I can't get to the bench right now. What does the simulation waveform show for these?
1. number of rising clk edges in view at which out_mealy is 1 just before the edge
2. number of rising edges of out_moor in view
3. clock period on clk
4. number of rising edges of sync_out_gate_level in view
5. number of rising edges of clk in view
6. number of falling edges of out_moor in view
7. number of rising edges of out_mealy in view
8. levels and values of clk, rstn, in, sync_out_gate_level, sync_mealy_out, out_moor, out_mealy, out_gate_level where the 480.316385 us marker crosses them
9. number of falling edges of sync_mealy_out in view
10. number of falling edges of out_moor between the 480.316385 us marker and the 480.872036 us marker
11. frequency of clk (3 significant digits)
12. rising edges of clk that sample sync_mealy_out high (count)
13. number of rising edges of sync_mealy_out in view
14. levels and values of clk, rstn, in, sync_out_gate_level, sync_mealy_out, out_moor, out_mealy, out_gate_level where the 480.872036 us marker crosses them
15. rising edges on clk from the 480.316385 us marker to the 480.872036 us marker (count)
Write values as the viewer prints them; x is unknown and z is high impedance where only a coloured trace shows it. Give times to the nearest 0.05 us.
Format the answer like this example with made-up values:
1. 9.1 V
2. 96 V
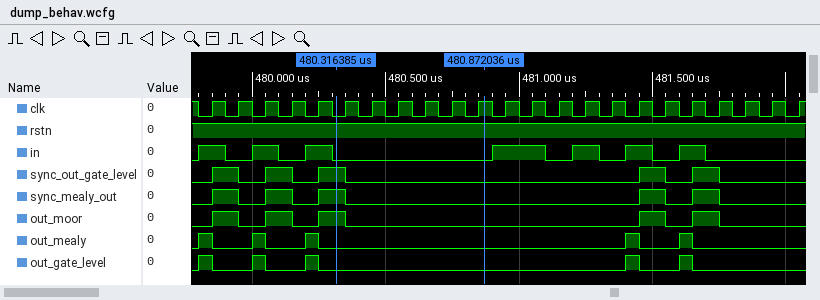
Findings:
1. 5
2. 5
3. 0.1 us
4. 5
5. 23
6. 5
7. 5
8. clk=0, rstn=1, in=0, sync_out_gate_level=1, sync_mealy_out=1, out_moor=1, out_mealy=0, out_gate_level=0
9. 5
10. 1
11. 10.0 MHz
12. 5
13. 5
14. clk=1, rstn=1, in=0, sync_out_gate_level=0, sync_mealy_out=0, out_moor=0, out_mealy=0, out_gate_level=0
15. 6
